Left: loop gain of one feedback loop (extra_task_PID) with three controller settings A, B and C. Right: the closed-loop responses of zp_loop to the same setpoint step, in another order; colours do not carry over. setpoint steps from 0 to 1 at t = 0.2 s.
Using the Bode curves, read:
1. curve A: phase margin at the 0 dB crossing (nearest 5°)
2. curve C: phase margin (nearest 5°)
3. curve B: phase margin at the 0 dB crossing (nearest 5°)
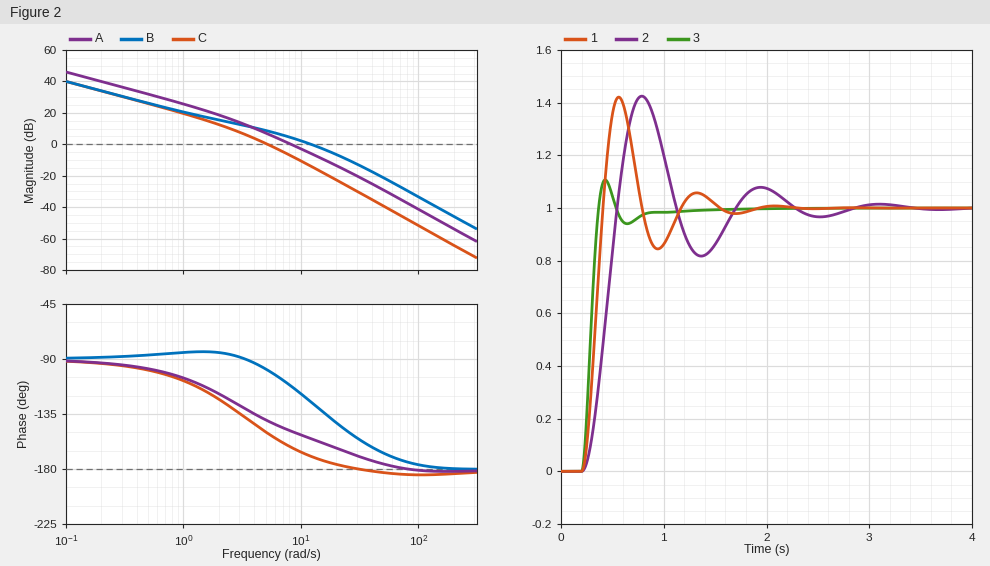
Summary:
30°
30°
55°
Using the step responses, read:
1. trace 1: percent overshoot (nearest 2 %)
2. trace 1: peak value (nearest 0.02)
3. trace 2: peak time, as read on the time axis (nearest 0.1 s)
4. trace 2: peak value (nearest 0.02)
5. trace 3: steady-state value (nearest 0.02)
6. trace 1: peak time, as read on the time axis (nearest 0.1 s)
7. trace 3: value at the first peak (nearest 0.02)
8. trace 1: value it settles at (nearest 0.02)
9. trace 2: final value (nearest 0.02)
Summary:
42 %
1.42
0.8 s
1.42
1.00
0.6 s
1.10
1.00
1.00
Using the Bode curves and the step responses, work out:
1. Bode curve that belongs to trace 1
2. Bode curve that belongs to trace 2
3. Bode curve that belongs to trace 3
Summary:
A
C
B
